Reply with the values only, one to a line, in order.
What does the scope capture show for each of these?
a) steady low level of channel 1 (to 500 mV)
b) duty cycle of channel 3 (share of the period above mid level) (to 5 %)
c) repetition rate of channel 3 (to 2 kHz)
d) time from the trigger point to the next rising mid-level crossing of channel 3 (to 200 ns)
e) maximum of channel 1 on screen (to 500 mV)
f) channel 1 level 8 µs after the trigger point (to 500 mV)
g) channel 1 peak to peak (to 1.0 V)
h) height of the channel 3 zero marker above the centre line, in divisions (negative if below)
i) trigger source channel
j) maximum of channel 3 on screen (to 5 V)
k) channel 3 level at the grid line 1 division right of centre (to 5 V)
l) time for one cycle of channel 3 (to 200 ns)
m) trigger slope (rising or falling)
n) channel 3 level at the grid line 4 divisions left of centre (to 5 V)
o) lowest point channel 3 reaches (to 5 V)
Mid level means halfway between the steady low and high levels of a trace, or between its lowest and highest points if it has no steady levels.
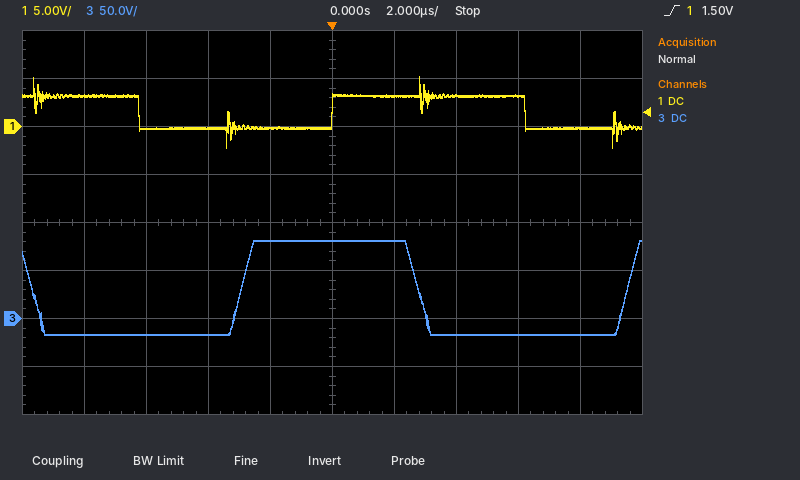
0.0 V
45 %
80 kHz
9.6 µs
5.0 V
0.0 V
7.0 V
-2.0 div
channel 1
80 V
80 V
12.4 µs
rising
-15 V
-15 V
